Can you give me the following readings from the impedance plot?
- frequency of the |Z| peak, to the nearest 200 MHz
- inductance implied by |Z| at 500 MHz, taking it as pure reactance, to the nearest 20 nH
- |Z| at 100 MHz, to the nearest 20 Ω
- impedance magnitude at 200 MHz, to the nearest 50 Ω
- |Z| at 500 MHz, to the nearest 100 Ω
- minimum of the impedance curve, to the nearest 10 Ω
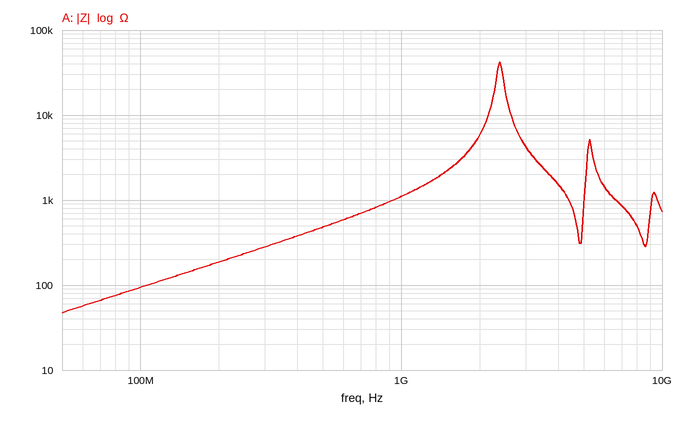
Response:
2.4 GHz
160 nH
100 Ω
200 Ω
500 Ω
50 Ω
